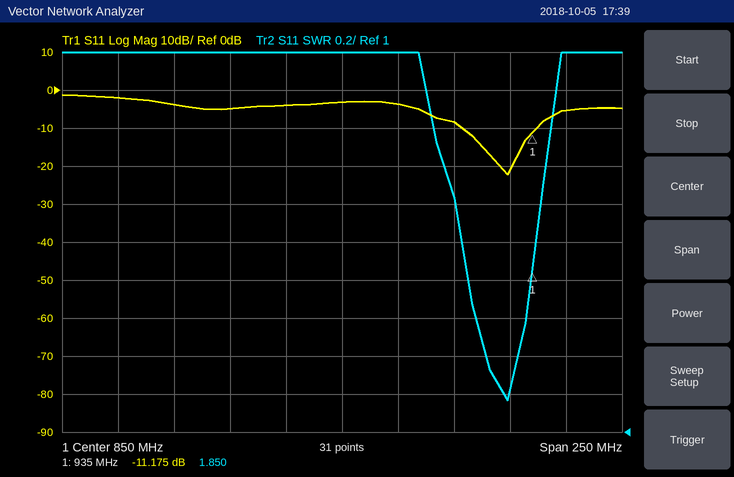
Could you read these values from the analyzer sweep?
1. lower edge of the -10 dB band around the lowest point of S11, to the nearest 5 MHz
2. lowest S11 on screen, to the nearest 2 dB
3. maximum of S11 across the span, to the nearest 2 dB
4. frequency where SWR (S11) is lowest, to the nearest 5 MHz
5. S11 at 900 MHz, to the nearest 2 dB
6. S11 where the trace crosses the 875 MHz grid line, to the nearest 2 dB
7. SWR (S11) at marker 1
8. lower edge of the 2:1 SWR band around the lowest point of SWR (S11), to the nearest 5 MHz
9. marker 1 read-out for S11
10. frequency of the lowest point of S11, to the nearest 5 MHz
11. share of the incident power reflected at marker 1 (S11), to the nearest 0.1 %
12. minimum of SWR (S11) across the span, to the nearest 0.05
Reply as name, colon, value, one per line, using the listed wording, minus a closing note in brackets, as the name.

lower edge of the -10 dB band around the lowest point of S11, to the nearest 5 MHz: 905 MHz
lowest S11 on screen, to the nearest 2 dB: -22 dB
maximum of S11 across the span, to the nearest 2 dB: -2 dB
frequency where SWR (S11) is lowest, to the nearest 5 MHz: 925 MHz
S11 at 900 MHz, to the nearest 2 dB: -8 dB
S11 where the trace crosses the 875 MHz grid line, to the nearest 2 dB: -4 dB
SWR (S11) at marker 1: 1.850
lower edge of the 2:1 SWR band around the lowest point of SWR (S11), to the nearest 5 MHz: 905 MHz
marker 1 read-out for S11: -11.175 dB
frequency of the lowest point of S11, to the nearest 5 MHz: 925 MHz
share of the incident power reflected at marker 1 (S11), to the nearest 0.1 %: 7.6 %
minimum of SWR (S11) across the span, to the nearest 0.05: 1.15
